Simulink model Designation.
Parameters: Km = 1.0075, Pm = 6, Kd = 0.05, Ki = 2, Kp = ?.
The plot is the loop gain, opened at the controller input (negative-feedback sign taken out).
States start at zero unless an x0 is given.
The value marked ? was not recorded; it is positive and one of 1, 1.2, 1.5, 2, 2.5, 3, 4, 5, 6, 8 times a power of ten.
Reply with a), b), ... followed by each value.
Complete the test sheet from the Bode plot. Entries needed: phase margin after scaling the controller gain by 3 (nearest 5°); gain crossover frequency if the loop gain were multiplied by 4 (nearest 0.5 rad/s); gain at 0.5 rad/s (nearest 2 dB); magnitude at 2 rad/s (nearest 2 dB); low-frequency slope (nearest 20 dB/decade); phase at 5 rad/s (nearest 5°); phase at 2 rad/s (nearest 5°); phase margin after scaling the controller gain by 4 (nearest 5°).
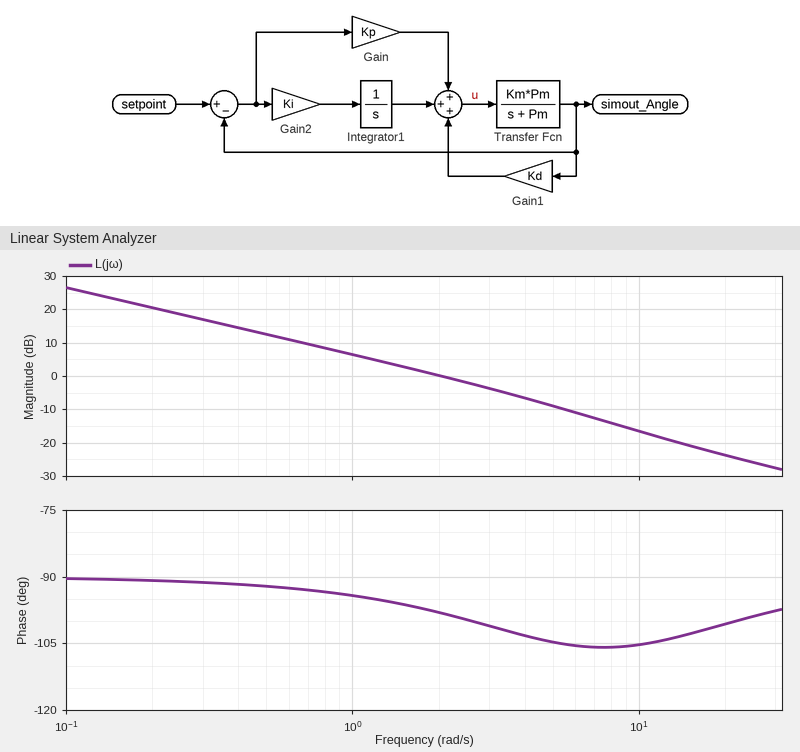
a) 75°
b) 6.5 rad/s
c) 12 dB
d) 0 dB
e) -20 dB/decade
f) -105°
g) -100°
h) 75°
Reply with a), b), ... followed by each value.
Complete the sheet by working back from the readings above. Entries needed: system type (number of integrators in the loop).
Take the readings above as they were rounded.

a) 1
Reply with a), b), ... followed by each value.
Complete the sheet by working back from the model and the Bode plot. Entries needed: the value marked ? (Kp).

a) 0.2
